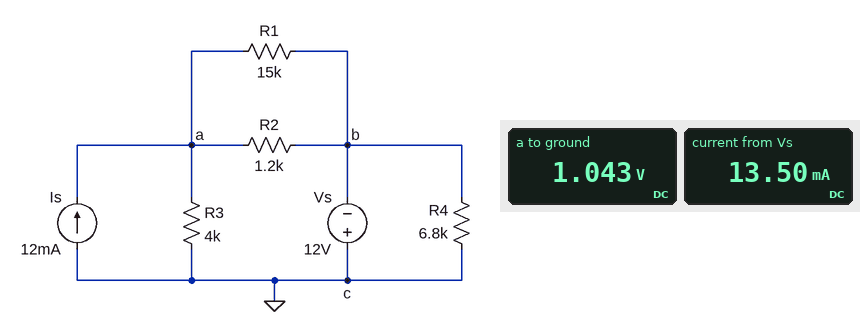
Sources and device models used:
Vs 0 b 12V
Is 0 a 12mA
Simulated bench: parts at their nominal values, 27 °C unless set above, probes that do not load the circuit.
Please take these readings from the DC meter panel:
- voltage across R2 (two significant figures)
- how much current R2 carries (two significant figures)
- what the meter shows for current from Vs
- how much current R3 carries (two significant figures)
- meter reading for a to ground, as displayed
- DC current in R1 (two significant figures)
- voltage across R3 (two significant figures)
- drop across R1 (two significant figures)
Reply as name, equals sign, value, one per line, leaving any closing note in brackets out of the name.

voltage across R2 = 13 V
how much current R2 carries = 11 mA
what the meter shows for current from Vs = 13.50 mA
how much current R3 carries = 260 µA
meter reading for a to ground, as displayed = 1.043 V
DC current in R1 = 870 µA
voltage across R3 = 1.0 V
drop across R1 = 13 V
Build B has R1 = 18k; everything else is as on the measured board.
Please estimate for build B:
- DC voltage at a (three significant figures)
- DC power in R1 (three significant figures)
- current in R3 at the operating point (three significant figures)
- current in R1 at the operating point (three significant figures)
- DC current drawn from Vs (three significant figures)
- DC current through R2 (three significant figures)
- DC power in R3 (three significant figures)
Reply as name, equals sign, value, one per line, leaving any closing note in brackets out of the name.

DC voltage at a = 1.17 V
DC power in R1 = 9.64 mW
current in R3 at the operating point = 293 µA
current in R1 at the operating point = 732 µA
DC current drawn from Vs = 13.5 mA
DC current through R2 = 11.0 mA
DC power in R3 = 343 µW
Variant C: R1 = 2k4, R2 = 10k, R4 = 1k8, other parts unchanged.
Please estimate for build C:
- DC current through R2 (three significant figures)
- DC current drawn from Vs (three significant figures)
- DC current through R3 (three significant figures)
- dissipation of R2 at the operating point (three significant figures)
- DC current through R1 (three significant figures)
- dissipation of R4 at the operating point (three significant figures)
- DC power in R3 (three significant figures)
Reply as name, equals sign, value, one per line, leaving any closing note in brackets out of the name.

DC current through R2 = 1.96 mA
DC current drawn from Vs = 16.8 mA
DC current through R3 = 1.89 mA
dissipation of R2 at the operating point = 38.3 mW
DC current through R1 = 8.15 mA
dissipation of R4 at the operating point = 80.0 mW
DC power in R3 = 14.3 mW
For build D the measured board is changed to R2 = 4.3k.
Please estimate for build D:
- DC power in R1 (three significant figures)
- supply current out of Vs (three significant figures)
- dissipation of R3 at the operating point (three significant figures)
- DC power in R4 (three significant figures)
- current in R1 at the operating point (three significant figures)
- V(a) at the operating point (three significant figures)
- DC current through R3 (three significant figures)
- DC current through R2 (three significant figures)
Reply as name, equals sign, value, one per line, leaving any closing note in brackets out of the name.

DC power in R1 = 49.7 mW
supply current out of Vs = 9.94 mA
dissipation of R3 at the operating point = 58.6 mW
DC power in R4 = 21.2 mW
current in R1 at the operating point = 1.82 mA
V(a) at the operating point = 15.3 V
DC current through R3 = 3.83 mA
DC current through R2 = 6.35 mA
